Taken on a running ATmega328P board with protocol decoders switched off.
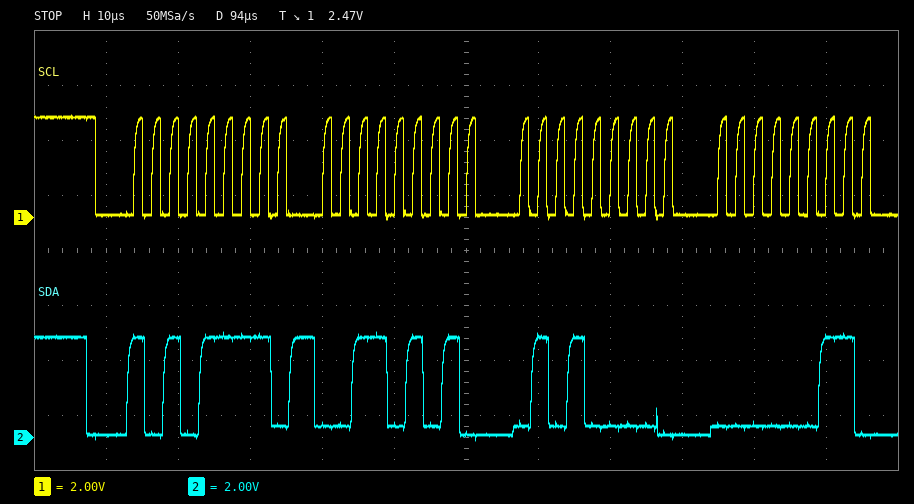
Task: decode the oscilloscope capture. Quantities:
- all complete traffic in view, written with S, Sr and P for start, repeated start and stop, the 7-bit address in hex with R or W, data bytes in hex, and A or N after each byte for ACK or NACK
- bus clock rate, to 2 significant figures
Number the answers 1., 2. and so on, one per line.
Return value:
1. S 57R A 35 A 50 A 03 A
2. 400 kHz
